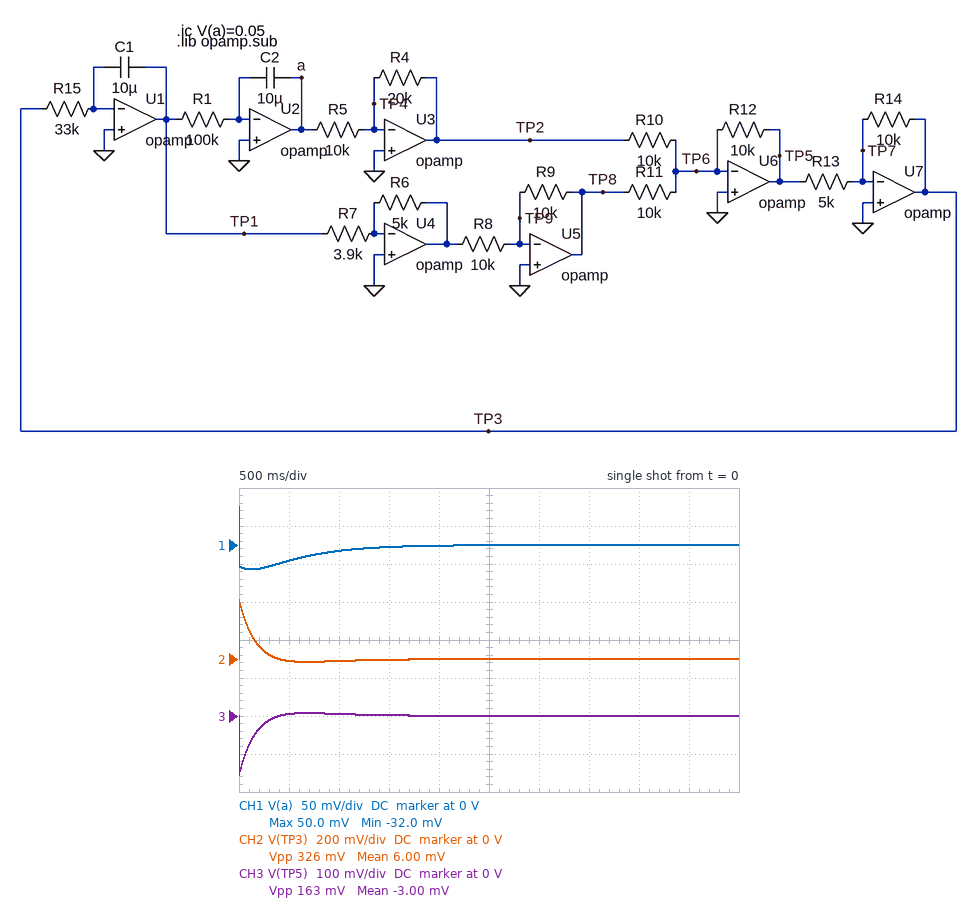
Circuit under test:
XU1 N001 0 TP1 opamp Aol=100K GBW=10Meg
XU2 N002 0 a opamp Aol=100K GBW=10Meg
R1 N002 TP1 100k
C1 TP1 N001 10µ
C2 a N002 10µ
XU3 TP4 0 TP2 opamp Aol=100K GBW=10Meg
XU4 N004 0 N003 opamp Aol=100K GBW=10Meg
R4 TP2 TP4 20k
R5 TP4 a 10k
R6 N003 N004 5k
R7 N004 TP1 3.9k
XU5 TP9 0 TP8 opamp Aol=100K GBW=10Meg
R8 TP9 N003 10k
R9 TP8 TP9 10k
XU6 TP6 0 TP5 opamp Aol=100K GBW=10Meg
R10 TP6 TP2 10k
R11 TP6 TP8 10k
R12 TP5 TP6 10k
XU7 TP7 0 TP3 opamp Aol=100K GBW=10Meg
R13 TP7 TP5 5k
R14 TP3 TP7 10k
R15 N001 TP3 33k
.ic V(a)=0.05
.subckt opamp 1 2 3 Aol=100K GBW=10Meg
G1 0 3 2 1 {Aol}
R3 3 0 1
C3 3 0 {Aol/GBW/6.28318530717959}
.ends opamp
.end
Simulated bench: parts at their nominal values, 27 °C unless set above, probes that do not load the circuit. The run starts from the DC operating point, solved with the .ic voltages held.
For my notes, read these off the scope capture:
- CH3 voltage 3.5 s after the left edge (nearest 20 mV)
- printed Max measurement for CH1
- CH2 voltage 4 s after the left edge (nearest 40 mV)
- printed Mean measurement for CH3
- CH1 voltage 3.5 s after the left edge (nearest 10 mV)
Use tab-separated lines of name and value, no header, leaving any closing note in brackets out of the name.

CH3 voltage 3.5 s after the left edge	0 V
printed Max measurement for CH1	50.0 mV
CH2 voltage 4 s after the left edge	0 V
printed Mean measurement for CH3	-3.00 mV
CH1 voltage 3.5 s after the left edge	0 V
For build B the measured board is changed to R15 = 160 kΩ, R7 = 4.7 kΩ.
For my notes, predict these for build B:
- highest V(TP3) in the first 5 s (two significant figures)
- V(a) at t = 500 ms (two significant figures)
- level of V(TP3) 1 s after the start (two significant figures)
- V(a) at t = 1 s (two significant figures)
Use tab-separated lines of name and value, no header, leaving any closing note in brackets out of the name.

highest V(TP3) in the first 5 s	380 mV
V(a) at t = 500 ms	-64 mV
level of V(TP3) 1 s after the start	71 mV
V(a) at t = 1 s	-47 mV
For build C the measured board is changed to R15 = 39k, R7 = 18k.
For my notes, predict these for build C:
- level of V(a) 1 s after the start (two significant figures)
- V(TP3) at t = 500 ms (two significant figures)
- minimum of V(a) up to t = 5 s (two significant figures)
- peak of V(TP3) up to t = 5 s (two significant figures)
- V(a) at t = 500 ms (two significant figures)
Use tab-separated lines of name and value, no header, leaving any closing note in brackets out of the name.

level of V(a) 1 s after the start	150 mV
V(TP3) at t = 500 ms	100 mV
minimum of V(a) up to t = 5 s	-330 mV
peak of V(TP3) up to t = 5 s	1.4 V
V(a) at t = 500 ms	-130 mV
